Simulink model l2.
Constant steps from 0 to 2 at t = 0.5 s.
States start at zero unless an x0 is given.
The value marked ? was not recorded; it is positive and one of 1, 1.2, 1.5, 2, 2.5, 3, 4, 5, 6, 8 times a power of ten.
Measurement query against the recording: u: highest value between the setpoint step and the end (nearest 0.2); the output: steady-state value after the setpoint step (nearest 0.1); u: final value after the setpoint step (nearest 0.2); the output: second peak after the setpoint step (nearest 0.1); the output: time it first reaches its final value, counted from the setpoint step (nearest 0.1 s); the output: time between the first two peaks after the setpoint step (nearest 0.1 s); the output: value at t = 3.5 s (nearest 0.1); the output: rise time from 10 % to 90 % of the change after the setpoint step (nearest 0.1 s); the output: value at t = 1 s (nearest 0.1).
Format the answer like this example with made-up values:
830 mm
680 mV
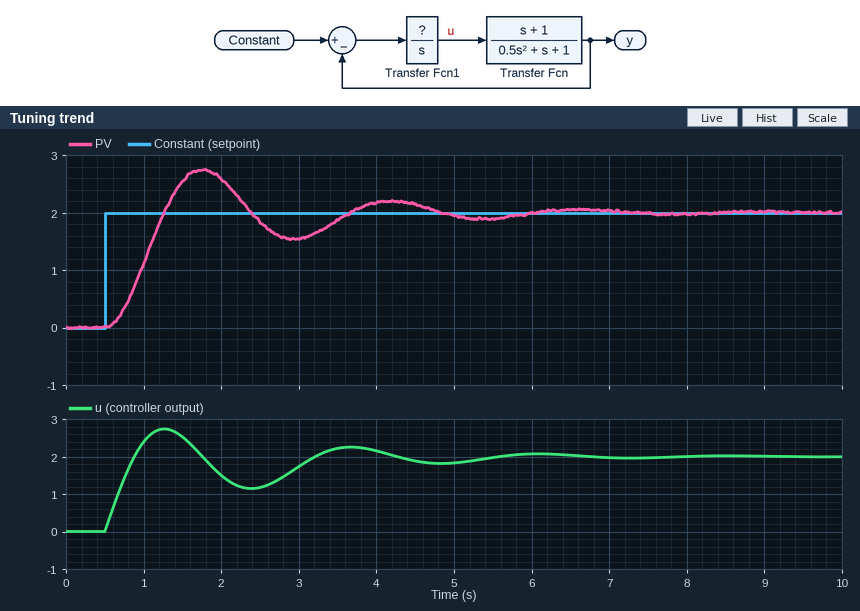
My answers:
2.8
2.0
2.0
2.2
0.8 s
2.4 s
1.9
0.5 s
1.1
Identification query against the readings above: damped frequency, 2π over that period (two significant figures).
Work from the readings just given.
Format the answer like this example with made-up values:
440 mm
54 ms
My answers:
2.6 rad/s
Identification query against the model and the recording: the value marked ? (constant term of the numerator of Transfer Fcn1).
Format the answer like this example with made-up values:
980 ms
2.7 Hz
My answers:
3
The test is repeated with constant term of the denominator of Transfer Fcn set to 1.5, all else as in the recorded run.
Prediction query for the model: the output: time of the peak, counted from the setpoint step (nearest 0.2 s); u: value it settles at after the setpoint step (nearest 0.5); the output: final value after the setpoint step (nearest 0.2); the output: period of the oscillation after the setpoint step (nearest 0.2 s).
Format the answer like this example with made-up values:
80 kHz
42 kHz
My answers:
1.2 s
3.0
2.0
2.2 s
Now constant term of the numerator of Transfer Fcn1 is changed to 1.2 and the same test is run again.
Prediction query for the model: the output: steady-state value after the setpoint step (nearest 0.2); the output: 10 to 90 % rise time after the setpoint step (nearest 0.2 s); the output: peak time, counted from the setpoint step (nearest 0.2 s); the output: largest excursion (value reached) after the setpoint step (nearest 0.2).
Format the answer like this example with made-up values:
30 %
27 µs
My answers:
2.0
1.0 s
2.0 s
2.2
